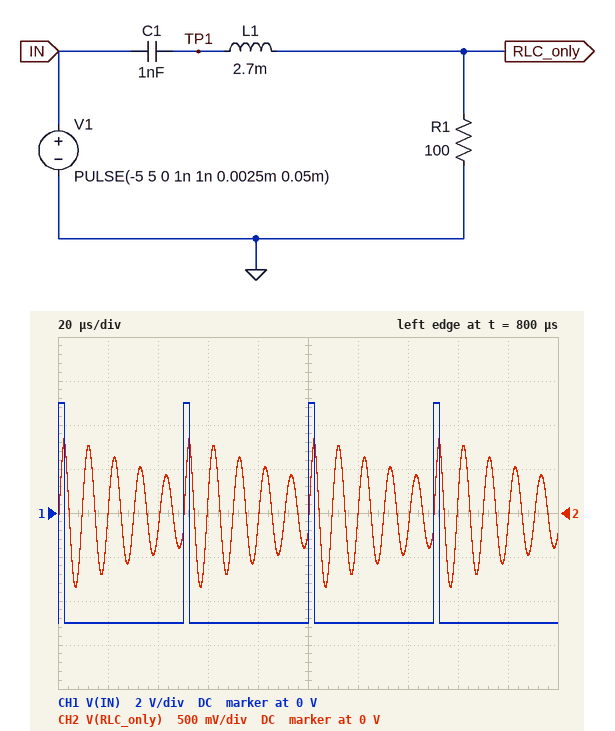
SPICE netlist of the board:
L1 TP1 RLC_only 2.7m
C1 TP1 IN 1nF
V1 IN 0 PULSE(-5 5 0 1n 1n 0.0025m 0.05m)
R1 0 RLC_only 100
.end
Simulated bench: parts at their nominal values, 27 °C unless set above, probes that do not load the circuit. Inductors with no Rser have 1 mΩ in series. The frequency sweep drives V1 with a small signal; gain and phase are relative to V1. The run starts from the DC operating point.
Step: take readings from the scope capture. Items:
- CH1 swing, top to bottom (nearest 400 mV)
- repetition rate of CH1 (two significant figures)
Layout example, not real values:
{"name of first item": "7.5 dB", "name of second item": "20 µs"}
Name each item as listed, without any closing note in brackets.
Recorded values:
{"CH1 swing, top to bottom": "10.0 V", "repetition rate of CH1": "20 kHz"}
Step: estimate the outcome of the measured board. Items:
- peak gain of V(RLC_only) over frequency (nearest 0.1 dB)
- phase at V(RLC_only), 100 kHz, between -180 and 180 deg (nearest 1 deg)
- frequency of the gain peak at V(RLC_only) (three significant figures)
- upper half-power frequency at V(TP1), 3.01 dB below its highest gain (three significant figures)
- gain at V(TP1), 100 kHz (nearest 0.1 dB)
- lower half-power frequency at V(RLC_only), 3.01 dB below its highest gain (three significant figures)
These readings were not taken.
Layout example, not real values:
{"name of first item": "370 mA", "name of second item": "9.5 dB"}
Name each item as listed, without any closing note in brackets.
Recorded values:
{"peak gain of V(RLC_only) over frequency": "0 dB", "phase at V(RLC_only), 100 kHz, between -180 and 180 deg": "-46 deg", "frequency of the gain peak at V(RLC_only)": "96.9 kHz", "upper half-power frequency at V(TP1), 3.01 dB below its highest gain": "100 kHz", "gain at V(TP1), 100 kHz": "21.4 dB", "lower half-power frequency at V(RLC_only), 3.01 dB below its highest gain": "94.0 kHz"}
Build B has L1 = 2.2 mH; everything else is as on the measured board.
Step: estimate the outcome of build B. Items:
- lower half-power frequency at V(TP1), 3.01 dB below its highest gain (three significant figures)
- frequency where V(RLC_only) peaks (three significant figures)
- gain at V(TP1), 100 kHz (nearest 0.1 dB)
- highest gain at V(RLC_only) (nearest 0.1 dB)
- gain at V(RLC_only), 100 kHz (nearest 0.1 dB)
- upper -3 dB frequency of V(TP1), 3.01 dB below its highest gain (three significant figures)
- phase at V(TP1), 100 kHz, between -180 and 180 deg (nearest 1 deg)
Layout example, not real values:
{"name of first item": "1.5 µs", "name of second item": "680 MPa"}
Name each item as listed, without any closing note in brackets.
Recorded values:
{"lower half-power frequency at V(TP1), 3.01 dB below its highest gain": "104 kHz", "frequency where V(RLC_only) peaks": "107 kHz", "gain at V(TP1), 100 kHz": "15.5 dB", "highest gain at V(RLC_only)": "0 dB", "gain at V(RLC_only), 100 kHz": "-7.3 dB", "upper -3 dB frequency of V(TP1), 3.01 dB below its highest gain": "111 kHz", "phase at V(TP1), 100 kHz, between -180 and 180 deg": "150 deg"}
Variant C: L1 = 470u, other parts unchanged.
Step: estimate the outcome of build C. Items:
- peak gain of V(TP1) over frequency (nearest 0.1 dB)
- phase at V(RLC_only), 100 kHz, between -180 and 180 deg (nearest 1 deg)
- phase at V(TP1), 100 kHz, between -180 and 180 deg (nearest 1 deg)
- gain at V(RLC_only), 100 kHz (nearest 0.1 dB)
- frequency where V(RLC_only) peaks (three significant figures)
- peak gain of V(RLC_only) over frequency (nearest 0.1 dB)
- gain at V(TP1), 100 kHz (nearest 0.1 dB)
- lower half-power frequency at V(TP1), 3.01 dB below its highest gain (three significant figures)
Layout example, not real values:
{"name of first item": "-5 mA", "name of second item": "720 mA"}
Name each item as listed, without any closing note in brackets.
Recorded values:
{"peak gain of V(TP1) over frequency": "16.8 dB", "phase at V(RLC_only), 100 kHz, between -180 and 180 deg": "86 deg", "phase at V(TP1), 100 kHz, between -180 and 180 deg": "157 deg", "gain at V(RLC_only), 100 kHz": "-22.3 dB", "frequency where V(RLC_only) peaks": "232 kHz", "peak gain of V(RLC_only) over frequency": "0 dB", "gain at V(TP1), 100 kHz": "-12.4 dB", "lower half-power frequency at V(TP1), 3.01 dB below its highest gain": "218 kHz"}
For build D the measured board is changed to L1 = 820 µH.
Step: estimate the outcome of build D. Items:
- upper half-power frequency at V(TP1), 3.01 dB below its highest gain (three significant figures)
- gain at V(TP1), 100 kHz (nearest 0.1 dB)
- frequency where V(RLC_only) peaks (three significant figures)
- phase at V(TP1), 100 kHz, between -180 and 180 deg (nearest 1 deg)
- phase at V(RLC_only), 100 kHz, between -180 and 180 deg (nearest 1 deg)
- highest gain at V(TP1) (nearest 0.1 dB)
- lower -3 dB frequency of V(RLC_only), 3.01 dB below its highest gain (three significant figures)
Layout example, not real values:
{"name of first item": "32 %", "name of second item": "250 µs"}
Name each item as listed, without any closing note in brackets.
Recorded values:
{"upper half-power frequency at V(TP1), 3.01 dB below its highest gain": "187 kHz", "gain at V(TP1), 100 kHz": "-6.3 dB", "frequency where V(RLC_only) peaks": "176 kHz", "phase at V(TP1), 100 kHz, between -180 and 180 deg": "164 deg", "phase at V(RLC_only), 100 kHz, between -180 and 180 deg": "85 deg", "highest gain at V(TP1)": "19.2 dB", "lower -3 dB frequency of V(RLC_only), 3.01 dB below its highest gain": "166 kHz"}
